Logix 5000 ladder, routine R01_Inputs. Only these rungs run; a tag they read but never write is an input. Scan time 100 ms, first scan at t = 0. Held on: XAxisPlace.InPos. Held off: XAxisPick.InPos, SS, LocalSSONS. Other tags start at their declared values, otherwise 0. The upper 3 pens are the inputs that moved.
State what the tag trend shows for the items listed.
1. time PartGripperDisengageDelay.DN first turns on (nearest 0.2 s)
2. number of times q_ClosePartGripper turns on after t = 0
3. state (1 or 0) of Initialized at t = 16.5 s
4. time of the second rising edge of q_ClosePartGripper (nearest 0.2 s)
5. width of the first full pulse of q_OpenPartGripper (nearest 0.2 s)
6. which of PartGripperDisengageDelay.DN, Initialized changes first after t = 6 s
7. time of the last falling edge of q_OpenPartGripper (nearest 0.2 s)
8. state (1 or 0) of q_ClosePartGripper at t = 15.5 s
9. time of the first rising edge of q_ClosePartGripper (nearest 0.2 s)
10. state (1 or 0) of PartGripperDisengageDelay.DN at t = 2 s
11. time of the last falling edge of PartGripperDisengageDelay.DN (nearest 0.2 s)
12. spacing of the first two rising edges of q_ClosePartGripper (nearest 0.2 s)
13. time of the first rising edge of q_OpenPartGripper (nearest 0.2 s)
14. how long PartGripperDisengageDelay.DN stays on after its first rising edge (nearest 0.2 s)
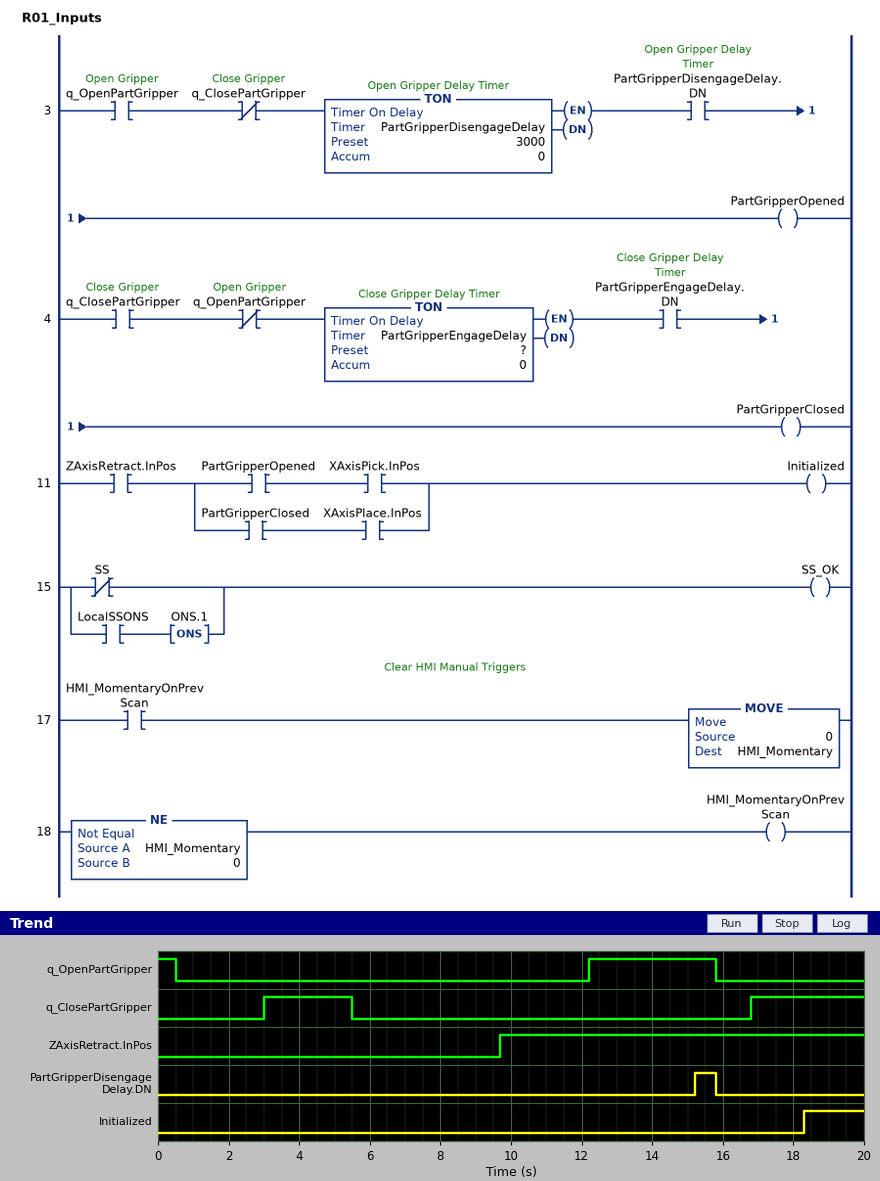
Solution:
15.2 s
2
0
16.8 s
3.6 s
PartGripperDisengageDelay.DN
15.8 s
0
3.0 s
0
15.8 s
13.8 s
12.2 s
0.6 s
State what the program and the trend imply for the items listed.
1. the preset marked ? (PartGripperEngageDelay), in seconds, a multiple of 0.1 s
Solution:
1.5 s
